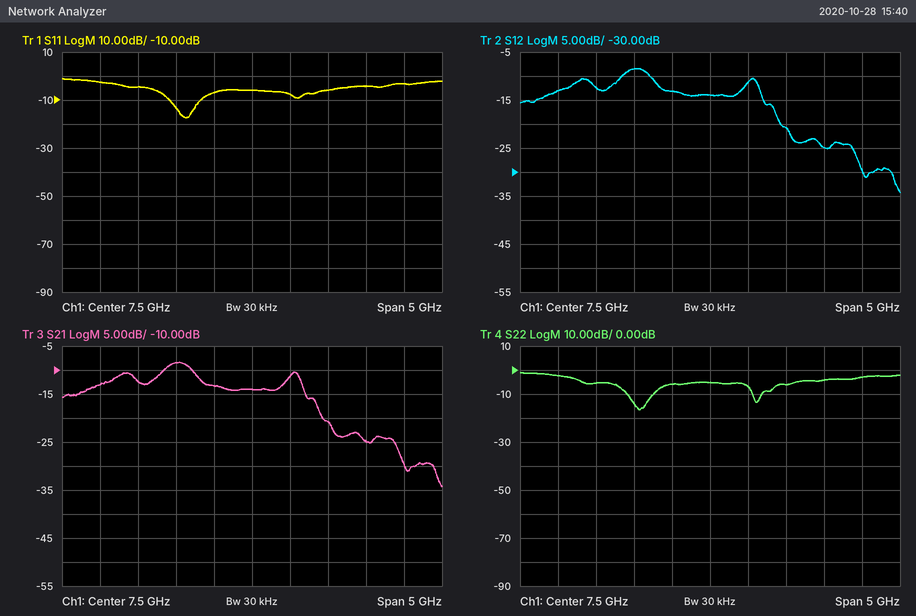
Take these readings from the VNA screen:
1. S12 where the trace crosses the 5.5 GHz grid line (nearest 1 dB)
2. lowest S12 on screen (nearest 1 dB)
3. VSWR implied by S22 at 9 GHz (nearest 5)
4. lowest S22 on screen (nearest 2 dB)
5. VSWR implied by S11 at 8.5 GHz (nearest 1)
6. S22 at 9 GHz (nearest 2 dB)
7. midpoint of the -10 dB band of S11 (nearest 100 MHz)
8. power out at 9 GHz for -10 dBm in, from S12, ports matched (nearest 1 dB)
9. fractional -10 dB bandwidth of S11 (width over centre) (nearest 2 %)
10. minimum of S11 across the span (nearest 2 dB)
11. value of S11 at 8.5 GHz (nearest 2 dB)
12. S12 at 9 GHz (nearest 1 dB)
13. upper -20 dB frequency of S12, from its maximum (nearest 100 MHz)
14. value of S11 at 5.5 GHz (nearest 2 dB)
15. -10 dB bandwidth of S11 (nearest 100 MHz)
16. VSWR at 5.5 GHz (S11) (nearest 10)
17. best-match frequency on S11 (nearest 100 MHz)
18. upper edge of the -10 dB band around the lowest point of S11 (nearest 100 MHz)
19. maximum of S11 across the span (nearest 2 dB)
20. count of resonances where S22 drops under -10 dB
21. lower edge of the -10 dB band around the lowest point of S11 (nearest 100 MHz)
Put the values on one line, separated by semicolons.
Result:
-13 dB; -34 dB; 5; -16 dB; 3; -4 dB; 6.6 GHz; -35 dBm; 6 %; -18 dB; -6 dB; -25 dB; 9.5 GHz; -2 dB; 400 MHz; 10; 6.6 GHz; 6.8 GHz; -2 dB; 2; 6.4 GHz
